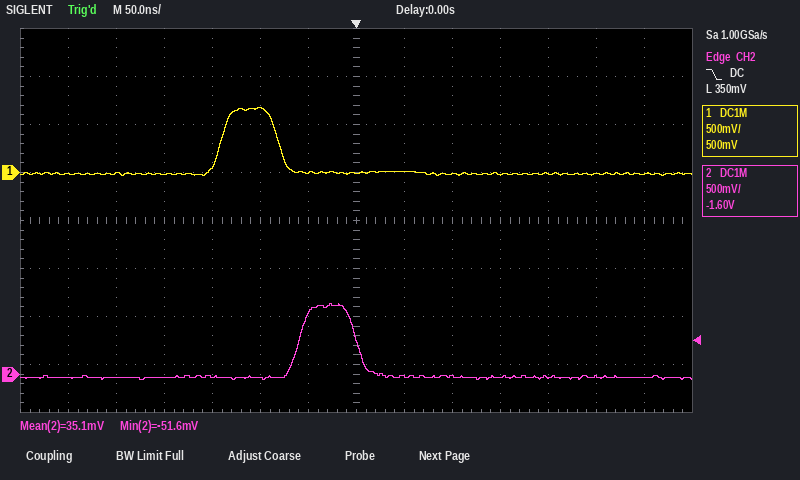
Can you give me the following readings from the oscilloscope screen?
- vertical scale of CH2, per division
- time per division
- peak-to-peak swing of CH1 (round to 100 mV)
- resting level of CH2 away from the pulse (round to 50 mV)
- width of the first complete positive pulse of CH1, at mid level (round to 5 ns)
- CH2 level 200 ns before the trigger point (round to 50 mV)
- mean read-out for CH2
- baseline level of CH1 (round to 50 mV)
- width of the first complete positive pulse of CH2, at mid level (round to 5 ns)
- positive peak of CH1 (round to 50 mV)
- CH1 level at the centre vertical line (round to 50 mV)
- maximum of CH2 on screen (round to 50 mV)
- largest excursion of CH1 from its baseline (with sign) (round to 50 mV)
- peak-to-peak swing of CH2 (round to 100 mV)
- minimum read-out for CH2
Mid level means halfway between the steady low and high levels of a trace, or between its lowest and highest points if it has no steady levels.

500 mV
50 ns
700 mV
-50 mV
60 ns
-50 mV
35.1 mV
0 mV
60 ns
700 mV
0 mV
750 mV
+700 mV
800 mV
-51.6 mV
